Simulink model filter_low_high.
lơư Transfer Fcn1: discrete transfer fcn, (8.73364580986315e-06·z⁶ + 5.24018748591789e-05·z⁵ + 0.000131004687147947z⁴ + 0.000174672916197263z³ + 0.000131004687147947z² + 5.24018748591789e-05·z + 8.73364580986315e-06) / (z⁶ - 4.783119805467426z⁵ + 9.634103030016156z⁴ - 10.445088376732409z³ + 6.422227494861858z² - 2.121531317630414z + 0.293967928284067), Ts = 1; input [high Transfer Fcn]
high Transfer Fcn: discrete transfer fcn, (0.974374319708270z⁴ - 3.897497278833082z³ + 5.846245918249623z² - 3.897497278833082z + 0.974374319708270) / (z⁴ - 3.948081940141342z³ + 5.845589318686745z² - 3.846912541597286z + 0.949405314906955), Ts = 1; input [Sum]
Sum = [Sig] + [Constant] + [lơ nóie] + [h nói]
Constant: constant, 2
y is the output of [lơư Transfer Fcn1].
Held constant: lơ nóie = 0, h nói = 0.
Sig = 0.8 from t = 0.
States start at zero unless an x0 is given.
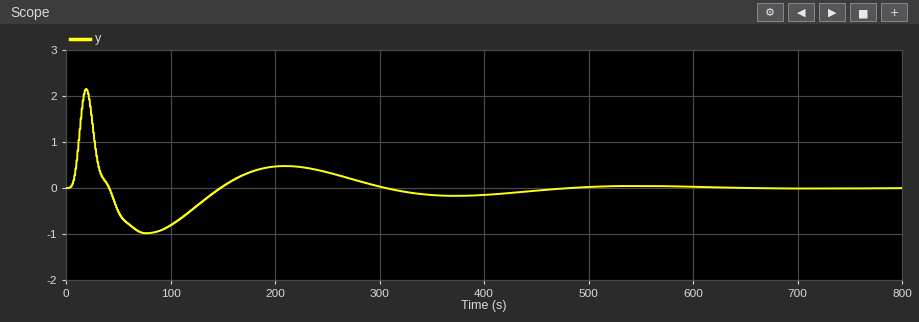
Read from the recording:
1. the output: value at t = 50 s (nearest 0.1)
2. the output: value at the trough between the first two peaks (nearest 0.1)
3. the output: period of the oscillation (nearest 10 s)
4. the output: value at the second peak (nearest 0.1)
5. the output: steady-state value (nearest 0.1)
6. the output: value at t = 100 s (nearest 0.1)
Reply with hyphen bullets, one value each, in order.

- -0.5
- -1.0
- 190 s
- 0.5
- 0.0
- -0.8
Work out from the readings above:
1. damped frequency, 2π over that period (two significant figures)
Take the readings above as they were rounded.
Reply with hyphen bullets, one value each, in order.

- 0.033 rad/s
